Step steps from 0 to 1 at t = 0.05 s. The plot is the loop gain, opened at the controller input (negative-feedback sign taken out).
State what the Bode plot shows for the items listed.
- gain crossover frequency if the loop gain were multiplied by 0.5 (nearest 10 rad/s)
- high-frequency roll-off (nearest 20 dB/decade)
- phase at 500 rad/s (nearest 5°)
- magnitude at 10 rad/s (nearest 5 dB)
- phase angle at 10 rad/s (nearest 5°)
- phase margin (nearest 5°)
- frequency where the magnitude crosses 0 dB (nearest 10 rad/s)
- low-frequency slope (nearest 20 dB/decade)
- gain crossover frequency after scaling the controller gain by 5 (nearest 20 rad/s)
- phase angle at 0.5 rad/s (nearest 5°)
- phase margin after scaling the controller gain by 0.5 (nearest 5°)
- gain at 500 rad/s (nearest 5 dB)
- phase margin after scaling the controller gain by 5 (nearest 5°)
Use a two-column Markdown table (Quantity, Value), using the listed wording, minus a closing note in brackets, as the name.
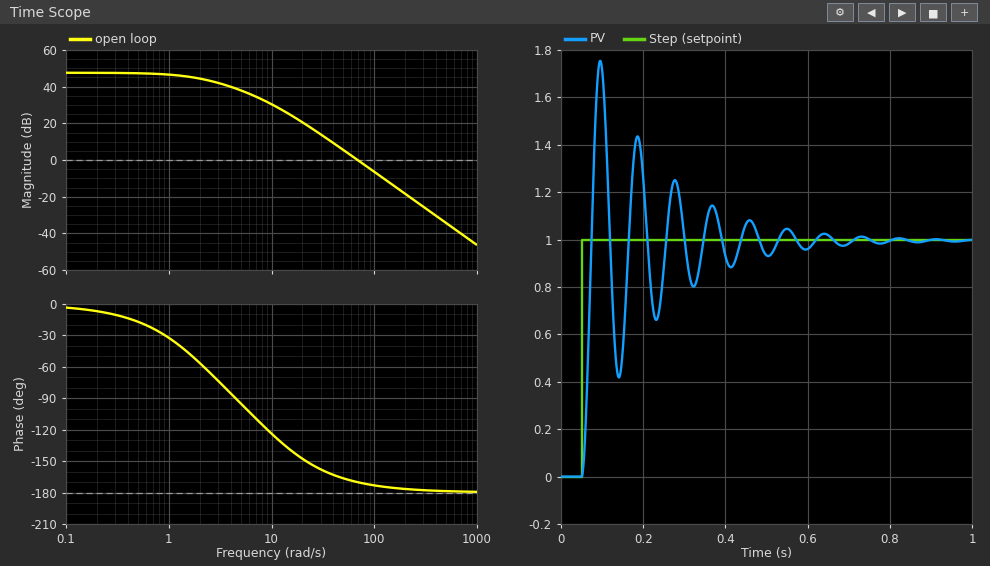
| Quantity | Value |
|---|---|
| gain crossover frequency if the loop gain were multiplied by 0.5 | 50 rad/s |
| high-frequency roll-off | -40 dB/decade |
| phase at 500 rad/s | -180° |
| magnitude at 10 rad/s | 30 dB |
| phase angle at 10 rad/s | -125° |
| phase margin | 10° |
| frequency where the magnitude crosses 0 dB | 70 rad/s |
| low-frequency slope | 0 dB/decade |
| gain crossover frequency after scaling the controller gain by 5 | 160 rad/s |
| phase angle at 0.5 rad/s | -15° |
| phase margin after scaling the controller gain by 0.5 | 15° |
| gain at 500 rad/s | -35 dB |
| phase margin after scaling the controller gain by 5 | 5° |
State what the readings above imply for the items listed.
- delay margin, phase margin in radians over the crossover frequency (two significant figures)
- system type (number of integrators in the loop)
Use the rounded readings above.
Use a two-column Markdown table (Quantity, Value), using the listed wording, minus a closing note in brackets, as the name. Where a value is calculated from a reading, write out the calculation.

| Quantity | Value |
|---|---|
| delay margin, phase margin in radians over the crossover frequency | 10 × π / 180 / 70 = 0.0025 s |
| system type | 0 |
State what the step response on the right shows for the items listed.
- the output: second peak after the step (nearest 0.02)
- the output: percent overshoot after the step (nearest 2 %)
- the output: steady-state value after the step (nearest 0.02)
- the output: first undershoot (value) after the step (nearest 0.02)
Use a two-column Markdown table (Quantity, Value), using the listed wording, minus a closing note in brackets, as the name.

| Quantity | Value |
|---|---|
| the output: second peak after the step | 1.44 |
| the output: percent overshoot after the step | 76 % |
| the output: steady-state value after the step | 1.00 |
| the output: first undershoot (value) after the step | 0.42 |
